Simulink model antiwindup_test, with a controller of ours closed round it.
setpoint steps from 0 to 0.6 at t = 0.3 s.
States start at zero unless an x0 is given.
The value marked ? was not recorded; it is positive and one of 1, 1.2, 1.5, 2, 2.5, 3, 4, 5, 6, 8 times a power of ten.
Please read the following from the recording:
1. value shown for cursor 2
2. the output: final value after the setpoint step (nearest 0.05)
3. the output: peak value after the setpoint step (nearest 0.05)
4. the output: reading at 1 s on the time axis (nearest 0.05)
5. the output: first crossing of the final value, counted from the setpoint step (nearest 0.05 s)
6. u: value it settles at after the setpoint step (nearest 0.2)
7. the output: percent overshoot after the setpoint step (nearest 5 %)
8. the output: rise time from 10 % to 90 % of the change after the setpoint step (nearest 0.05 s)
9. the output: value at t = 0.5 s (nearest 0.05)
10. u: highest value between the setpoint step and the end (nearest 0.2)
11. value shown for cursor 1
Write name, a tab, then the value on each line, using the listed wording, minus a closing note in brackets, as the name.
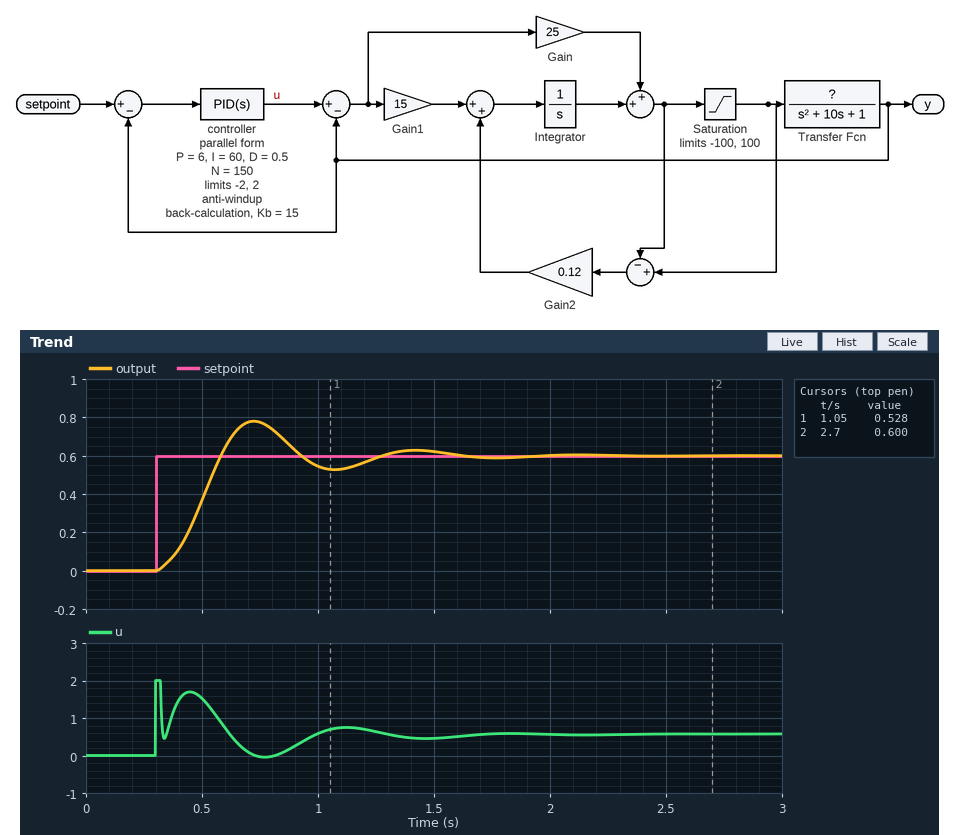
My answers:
value shown for cursor 2	0.600
the output: final value after the setpoint step	0.60
the output: peak value after the setpoint step	0.80
the output: reading at 1 s on the time axis	0.55
the output: first crossing of the final value, counted from the setpoint step	0.30 s
u: value it settles at after the setpoint step	0.6
the output: percent overshoot after the setpoint step	30 %
the output: rise time from 10 % to 90 % of the change after the setpoint step	0.20 s
the output: value at t = 0.5 s	0.35
u: highest value between the setpoint step and the end	2.0
value shown for cursor 1	0.528
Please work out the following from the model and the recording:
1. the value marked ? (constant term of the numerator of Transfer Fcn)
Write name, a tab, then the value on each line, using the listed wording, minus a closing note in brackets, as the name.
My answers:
the value marked ?	1
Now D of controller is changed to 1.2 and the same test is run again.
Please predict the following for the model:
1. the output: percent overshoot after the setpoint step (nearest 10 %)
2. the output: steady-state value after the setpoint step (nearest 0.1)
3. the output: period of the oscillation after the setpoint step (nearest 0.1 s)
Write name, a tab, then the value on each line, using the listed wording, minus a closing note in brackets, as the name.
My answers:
the output: percent overshoot after the setpoint step	40 %
the output: steady-state value after the setpoint step	0.6
the output: period of the oscillation after the setpoint step	1.0 s
